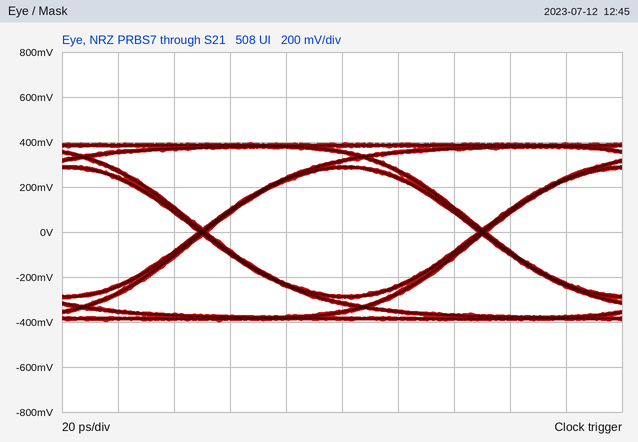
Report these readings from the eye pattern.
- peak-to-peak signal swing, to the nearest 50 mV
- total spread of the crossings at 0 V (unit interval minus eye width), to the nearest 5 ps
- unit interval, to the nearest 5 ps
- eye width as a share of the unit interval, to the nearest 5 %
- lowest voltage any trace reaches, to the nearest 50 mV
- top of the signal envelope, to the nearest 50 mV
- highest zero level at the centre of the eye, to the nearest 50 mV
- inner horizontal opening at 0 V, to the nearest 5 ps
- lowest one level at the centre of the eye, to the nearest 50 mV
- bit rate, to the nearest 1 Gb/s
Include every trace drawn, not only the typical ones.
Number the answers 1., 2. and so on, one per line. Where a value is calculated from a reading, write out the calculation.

1. 800 mV
2. 5 ps
3. 100 ps
4. 95 ps / 100 ps ≈ 95 %
5. -400 mV
6. 400 mV
7. -300 mV
8. 95 ps
9. 300 mV
10. 10 Gb/s
